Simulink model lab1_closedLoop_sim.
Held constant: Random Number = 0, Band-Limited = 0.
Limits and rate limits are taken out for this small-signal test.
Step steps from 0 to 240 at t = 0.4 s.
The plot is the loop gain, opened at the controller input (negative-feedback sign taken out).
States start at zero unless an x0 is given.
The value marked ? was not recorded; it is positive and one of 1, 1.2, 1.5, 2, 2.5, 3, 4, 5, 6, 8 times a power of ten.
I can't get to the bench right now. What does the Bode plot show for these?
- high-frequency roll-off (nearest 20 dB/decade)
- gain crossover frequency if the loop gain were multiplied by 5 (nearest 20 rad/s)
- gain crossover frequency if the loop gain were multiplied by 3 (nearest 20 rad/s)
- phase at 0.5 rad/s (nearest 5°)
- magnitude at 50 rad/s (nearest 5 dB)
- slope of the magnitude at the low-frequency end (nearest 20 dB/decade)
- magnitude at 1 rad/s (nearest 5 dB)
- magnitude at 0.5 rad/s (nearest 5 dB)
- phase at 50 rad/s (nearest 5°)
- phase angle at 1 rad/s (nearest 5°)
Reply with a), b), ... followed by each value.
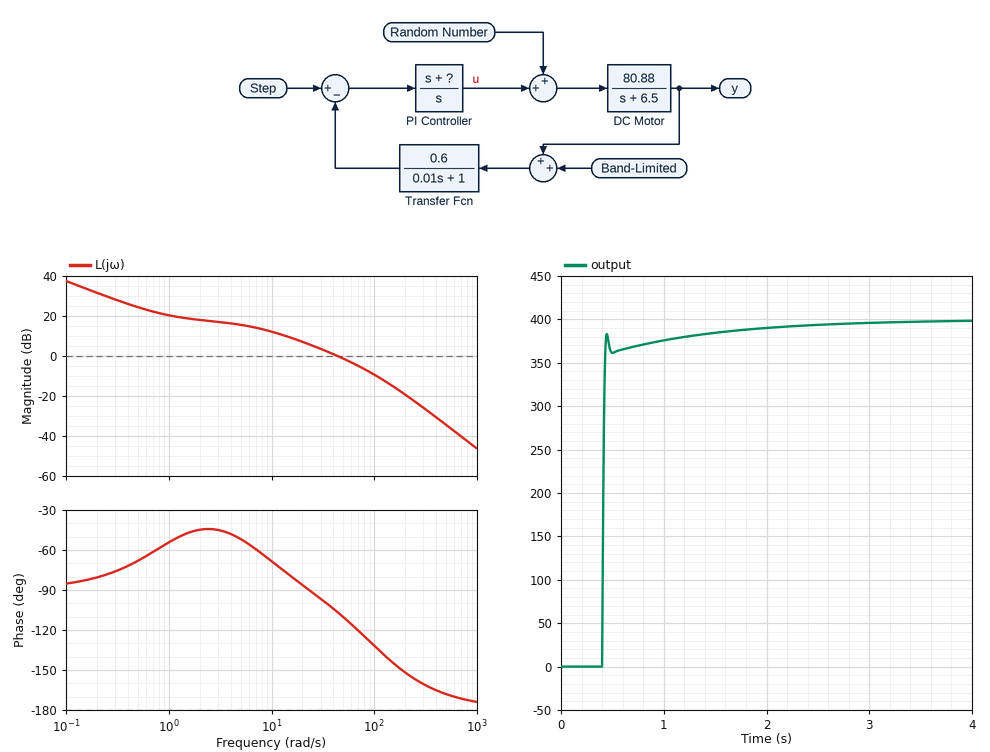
a) -40 dB/decade
b) 140 rad/s
c) 100 rad/s
d) -70°
e) 0 dB
f) -20 dB/decade
g) 20 dB
h) 25 dB
i) -110°
j) -55°
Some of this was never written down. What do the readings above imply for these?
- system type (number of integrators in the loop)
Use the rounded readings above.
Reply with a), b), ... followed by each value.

a) 1
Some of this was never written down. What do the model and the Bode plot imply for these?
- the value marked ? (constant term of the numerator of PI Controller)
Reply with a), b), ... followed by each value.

a) 1
